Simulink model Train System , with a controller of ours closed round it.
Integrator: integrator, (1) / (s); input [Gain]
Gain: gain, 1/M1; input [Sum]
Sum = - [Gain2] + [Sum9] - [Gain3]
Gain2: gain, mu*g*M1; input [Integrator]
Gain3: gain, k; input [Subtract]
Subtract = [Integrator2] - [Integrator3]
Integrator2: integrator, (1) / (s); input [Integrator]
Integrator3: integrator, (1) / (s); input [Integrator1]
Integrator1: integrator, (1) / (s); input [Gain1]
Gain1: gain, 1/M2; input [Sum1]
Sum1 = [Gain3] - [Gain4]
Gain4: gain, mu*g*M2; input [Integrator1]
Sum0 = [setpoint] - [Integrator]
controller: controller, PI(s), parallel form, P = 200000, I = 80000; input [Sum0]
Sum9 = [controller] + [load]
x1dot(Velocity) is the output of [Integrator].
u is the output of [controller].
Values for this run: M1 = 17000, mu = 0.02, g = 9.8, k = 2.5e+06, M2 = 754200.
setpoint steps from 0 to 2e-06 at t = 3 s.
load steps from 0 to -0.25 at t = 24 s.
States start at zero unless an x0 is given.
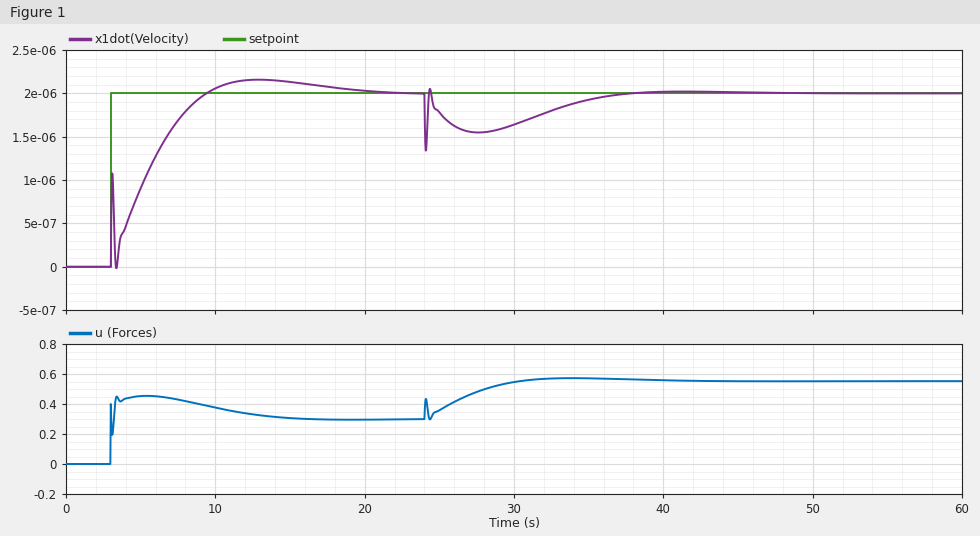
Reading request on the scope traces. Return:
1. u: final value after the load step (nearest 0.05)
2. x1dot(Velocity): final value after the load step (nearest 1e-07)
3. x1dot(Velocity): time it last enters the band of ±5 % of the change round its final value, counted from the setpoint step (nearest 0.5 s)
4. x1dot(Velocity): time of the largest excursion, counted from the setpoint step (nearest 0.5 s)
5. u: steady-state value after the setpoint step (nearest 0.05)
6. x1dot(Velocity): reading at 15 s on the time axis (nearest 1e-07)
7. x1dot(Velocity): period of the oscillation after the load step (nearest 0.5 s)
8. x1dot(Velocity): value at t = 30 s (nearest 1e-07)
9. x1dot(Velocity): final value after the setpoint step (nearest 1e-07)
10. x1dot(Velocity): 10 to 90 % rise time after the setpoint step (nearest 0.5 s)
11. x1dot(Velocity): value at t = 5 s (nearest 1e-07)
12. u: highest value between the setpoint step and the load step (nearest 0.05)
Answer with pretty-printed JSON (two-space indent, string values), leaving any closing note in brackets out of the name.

{
  "u: final value after the load step": "0.55",
  "x1dot(Velocity): final value after the load step": "0.0000020",
  "x1dot(Velocity): time it last enters the band of ±5 % of the change round its final value, counted from the setpoint step": "13.5 s",
  "x1dot(Velocity): time of the largest excursion, counted from the setpoint step": "10.0 s",
  "u: steady-state value after the setpoint step": "0.30",
  "x1dot(Velocity): reading at 15 s on the time axis": "0.0000021",
  "x1dot(Velocity): period of the oscillation after the load step": "3.5 s",
  "x1dot(Velocity): value at t = 30 s": "0.0000016",
  "x1dot(Velocity): final value after the setpoint step": "0.0000020",
  "x1dot(Velocity): 10 to 90 % rise time after the setpoint step": "5.0 s",
  "x1dot(Velocity): value at t = 5 s": "0.0000009",
  "u: highest value between the setpoint step and the load step": "0.45"
}
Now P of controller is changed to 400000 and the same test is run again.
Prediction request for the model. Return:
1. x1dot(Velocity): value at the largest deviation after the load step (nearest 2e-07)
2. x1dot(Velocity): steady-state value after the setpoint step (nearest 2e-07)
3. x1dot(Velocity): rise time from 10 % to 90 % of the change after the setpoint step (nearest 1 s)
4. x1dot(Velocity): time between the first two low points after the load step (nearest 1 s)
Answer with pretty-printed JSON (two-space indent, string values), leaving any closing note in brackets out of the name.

{
  "x1dot(Velocity): value at the largest deviation after the load step": "0.0000016",
  "x1dot(Velocity): steady-state value after the setpoint step": "0.0000020",
  "x1dot(Velocity): rise time from 10 % to 90 % of the change after the setpoint step": "4 s",
  "x1dot(Velocity): time between the first two low points after the load step": "3 s"
}
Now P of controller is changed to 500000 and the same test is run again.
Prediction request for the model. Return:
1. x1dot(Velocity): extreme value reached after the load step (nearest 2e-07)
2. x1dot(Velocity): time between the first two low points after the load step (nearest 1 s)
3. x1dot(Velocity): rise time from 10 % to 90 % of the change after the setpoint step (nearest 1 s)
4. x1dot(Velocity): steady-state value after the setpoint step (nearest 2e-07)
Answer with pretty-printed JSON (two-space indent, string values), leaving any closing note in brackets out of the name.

{
  "x1dot(Velocity): extreme value reached after the load step": "0.0000016",
  "x1dot(Velocity): time between the first two low points after the load step": "3 s",
  "x1dot(Velocity): rise time from 10 % to 90 % of the change after the setpoint step": "4 s",
  "x1dot(Velocity): steady-state value after the setpoint step": "0.0000020"
}
